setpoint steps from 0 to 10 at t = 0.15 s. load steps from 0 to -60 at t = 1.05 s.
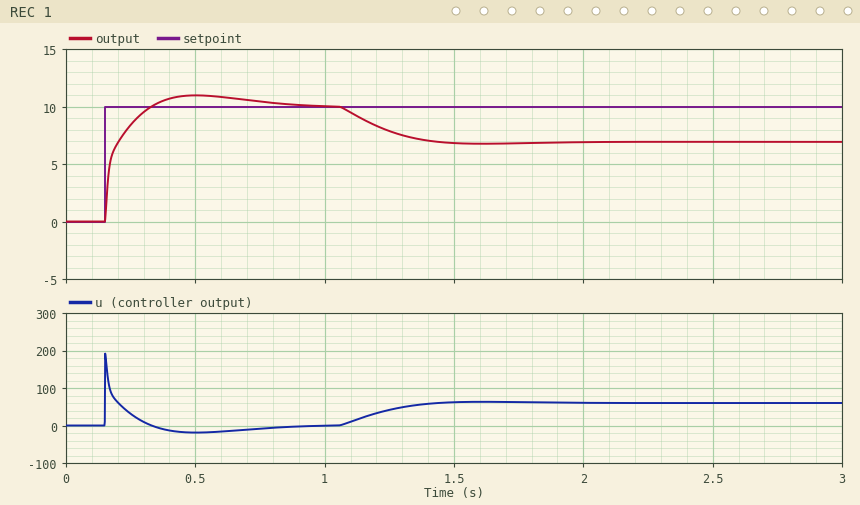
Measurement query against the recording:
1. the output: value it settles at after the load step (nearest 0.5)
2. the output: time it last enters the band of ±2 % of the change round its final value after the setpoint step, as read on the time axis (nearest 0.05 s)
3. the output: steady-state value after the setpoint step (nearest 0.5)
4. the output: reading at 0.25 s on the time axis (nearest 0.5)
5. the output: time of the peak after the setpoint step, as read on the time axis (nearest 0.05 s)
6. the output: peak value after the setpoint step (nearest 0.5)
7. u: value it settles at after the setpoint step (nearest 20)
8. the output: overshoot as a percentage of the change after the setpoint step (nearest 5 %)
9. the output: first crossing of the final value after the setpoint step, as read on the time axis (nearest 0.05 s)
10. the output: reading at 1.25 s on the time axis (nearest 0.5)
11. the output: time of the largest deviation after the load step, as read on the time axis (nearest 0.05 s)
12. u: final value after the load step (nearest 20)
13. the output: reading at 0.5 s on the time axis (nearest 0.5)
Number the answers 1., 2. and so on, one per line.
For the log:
1. 7.0
2. 0.85 s
3. 10.0
4. 8.5
5. 0.50 s
6. 11.0
7. 0
8. 10 %
9. 0.35 s
10. 8.0
11. 1.60 s
12. 60
13. 11.0
